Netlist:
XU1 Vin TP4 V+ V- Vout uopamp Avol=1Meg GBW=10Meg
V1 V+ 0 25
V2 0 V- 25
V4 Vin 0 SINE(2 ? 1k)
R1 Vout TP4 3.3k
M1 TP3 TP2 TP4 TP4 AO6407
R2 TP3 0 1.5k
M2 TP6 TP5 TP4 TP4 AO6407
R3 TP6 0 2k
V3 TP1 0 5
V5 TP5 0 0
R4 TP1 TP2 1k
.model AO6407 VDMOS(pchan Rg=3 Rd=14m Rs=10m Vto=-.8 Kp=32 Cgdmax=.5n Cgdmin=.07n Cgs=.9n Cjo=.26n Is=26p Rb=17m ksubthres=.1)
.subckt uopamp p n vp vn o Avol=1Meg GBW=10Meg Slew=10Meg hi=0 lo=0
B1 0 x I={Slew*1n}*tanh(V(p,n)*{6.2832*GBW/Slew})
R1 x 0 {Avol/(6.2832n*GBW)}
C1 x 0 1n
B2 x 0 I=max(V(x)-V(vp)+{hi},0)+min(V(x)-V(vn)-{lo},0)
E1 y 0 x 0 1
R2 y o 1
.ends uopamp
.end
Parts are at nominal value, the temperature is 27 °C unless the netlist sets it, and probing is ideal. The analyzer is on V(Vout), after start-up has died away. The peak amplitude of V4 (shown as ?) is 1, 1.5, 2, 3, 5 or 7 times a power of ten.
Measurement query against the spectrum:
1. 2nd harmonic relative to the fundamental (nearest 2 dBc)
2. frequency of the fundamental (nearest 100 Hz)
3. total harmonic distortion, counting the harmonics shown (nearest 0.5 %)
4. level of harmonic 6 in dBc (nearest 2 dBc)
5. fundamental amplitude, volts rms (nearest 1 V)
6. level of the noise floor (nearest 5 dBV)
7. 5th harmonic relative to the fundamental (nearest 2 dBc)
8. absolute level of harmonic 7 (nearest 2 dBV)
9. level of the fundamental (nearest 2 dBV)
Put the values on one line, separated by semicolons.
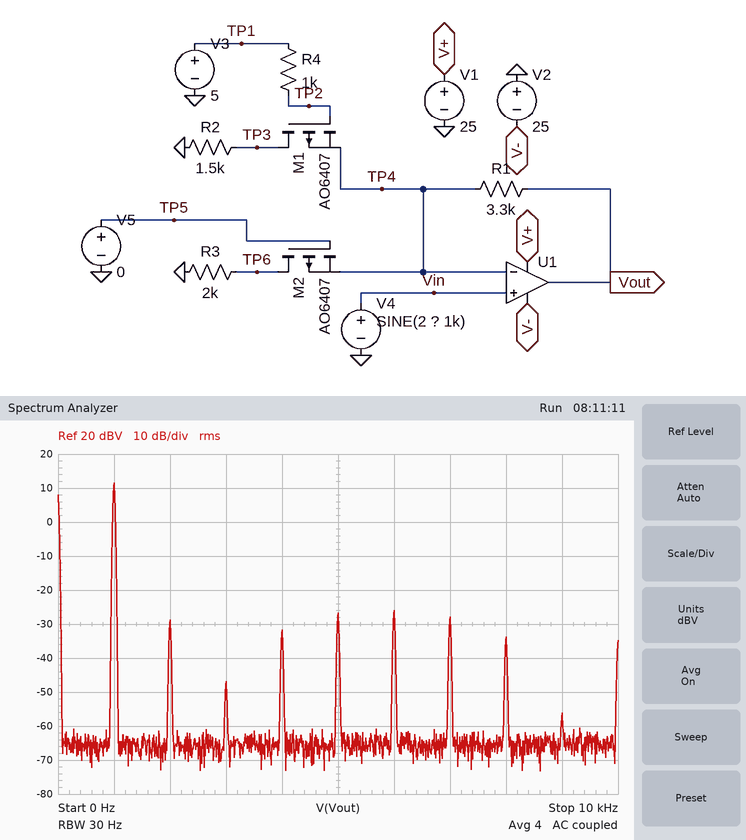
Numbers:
-40 dBc; 1.0 kHz; 2.5 %; -38 dBc; 4 V; -65 dBV; -38 dBc; -28 dBV; 12 dBV
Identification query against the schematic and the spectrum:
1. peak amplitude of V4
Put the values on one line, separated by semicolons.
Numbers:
2 V
